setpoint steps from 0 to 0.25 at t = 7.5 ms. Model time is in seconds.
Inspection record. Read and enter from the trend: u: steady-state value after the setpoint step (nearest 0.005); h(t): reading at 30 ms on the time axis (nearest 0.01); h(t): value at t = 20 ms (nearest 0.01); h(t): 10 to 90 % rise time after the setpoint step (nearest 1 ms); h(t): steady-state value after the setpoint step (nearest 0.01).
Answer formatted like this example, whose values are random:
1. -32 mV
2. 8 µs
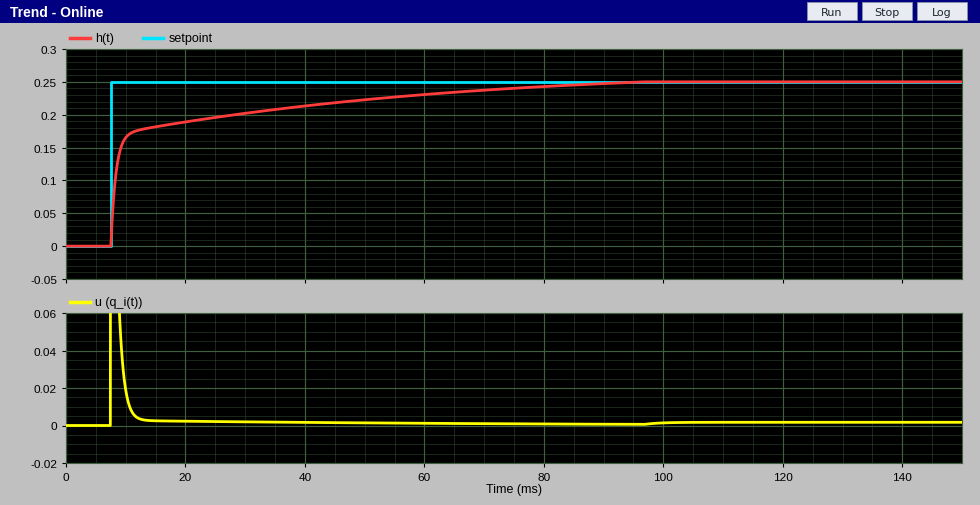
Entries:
1. 0.000
2. 0.20
3. 0.19
4. 45 ms
5. 0.25
